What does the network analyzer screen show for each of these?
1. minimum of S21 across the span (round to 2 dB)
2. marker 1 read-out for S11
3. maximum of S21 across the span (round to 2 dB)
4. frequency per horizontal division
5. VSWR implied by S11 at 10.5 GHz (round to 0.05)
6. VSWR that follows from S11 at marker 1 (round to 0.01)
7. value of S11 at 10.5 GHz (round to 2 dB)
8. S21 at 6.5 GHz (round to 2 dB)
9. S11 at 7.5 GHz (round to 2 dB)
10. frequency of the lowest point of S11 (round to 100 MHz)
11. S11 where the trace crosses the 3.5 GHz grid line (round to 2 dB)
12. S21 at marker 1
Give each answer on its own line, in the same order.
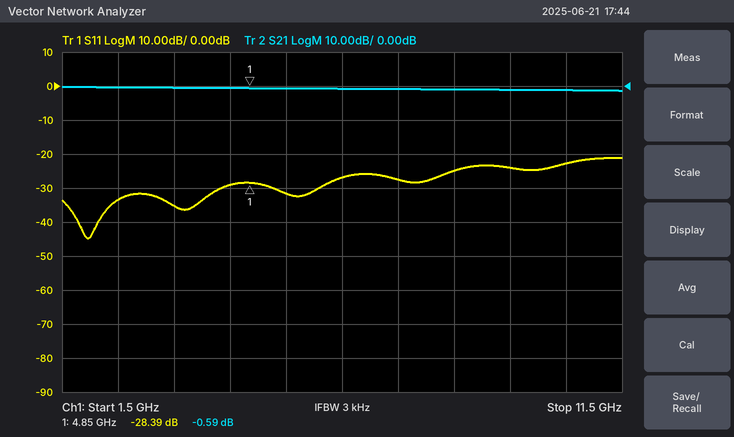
-2 dB
-28.39 dB
0 dB
1 GHz
1.15
1.08
-22 dB
0 dB
-28 dB
2.0 GHz
-36 dB
-0.59 dB
